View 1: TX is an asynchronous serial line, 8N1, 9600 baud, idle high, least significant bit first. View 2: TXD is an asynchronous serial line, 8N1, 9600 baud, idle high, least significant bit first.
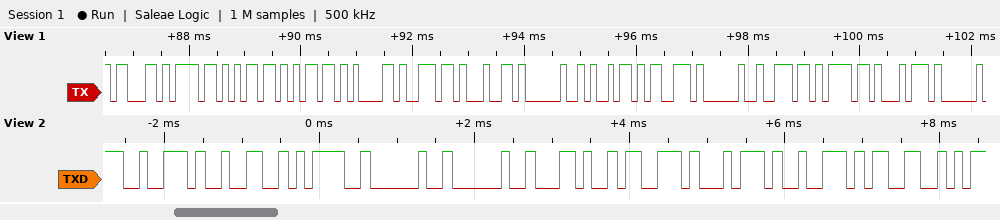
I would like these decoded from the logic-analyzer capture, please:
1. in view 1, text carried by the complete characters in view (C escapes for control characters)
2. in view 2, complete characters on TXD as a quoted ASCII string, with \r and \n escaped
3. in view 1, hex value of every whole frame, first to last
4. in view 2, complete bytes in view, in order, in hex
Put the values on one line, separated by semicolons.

"command is not"; "r2=  ,str3"; 63 6F 6D 6D 61 6E 64 20 69 73 20 6E 6F 74; 72 32 3D 20 20 2C 73 74 72 33
